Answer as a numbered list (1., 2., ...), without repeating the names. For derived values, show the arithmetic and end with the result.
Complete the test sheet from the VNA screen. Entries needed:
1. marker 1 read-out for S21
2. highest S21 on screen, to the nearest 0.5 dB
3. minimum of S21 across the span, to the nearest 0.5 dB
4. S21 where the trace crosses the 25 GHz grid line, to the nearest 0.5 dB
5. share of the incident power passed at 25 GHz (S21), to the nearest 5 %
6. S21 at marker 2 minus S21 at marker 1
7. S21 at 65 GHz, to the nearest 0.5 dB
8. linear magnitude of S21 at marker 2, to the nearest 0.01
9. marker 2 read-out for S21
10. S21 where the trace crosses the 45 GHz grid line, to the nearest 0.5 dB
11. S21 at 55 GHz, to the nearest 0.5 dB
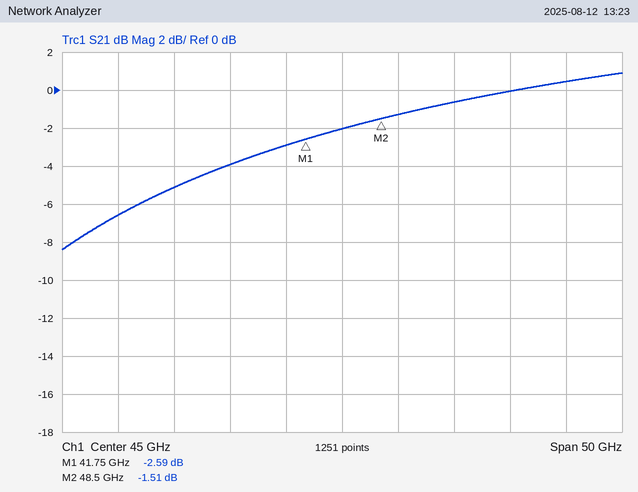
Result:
1. -2.59 dB
2. 1.0 dB
3. -8.5 dB
4. -6.5 dB
5. 10^(-6.5/10) ≈ 22.4 %, so 20 % to the nearest 5 %
6. -1.51 − (-2.59) = 1.08 dB
7. 0.5 dB
8. 10^(-1.51/20) ≈ 0.84
9. -1.51 dB
10. -2.0 dB
11. -0.5 dB
